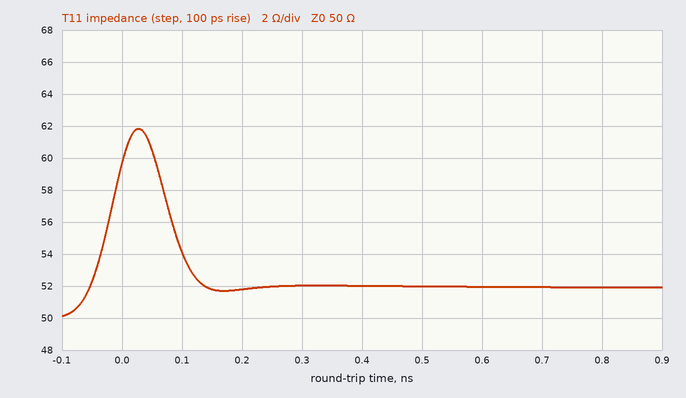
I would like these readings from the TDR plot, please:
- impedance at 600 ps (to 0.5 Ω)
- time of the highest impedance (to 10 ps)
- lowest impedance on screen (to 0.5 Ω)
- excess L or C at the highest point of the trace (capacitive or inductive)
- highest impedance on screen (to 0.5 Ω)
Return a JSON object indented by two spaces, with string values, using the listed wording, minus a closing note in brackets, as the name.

{
  "impedance at 600 ps": "52.0 Ω",
  "time of the highest impedance": "30 ps",
  "lowest impedance on screen": "50.0 Ω",
  "excess L or C at the highest point of the trace": "inductive",
  "highest impedance on screen": "62.0 Ω"
}
